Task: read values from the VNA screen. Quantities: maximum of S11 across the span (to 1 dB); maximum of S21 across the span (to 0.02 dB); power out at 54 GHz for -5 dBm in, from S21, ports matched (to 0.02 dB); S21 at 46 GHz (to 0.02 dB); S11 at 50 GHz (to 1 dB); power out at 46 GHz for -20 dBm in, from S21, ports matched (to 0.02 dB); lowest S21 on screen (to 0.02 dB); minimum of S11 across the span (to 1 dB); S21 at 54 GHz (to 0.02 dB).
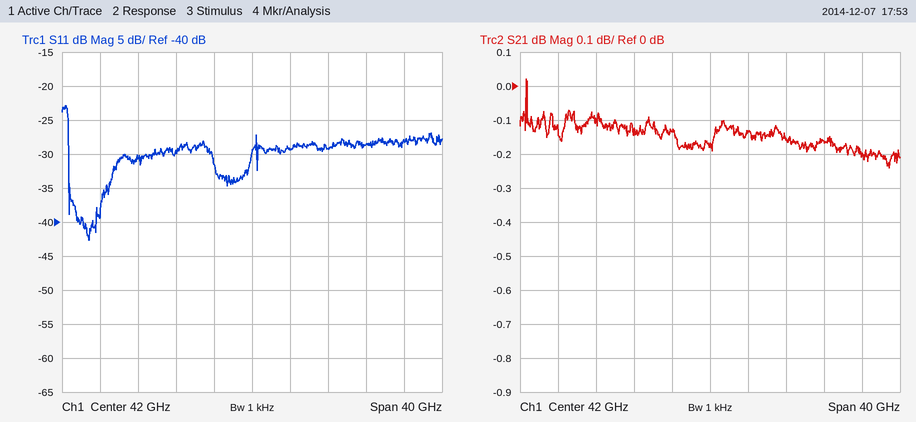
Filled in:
-23 dB
0.02 dB
-5.16 dBm
-0.14 dB
-29 dB
-20.14 dBm
-0.24 dB
-43 dB
-0.16 dB
